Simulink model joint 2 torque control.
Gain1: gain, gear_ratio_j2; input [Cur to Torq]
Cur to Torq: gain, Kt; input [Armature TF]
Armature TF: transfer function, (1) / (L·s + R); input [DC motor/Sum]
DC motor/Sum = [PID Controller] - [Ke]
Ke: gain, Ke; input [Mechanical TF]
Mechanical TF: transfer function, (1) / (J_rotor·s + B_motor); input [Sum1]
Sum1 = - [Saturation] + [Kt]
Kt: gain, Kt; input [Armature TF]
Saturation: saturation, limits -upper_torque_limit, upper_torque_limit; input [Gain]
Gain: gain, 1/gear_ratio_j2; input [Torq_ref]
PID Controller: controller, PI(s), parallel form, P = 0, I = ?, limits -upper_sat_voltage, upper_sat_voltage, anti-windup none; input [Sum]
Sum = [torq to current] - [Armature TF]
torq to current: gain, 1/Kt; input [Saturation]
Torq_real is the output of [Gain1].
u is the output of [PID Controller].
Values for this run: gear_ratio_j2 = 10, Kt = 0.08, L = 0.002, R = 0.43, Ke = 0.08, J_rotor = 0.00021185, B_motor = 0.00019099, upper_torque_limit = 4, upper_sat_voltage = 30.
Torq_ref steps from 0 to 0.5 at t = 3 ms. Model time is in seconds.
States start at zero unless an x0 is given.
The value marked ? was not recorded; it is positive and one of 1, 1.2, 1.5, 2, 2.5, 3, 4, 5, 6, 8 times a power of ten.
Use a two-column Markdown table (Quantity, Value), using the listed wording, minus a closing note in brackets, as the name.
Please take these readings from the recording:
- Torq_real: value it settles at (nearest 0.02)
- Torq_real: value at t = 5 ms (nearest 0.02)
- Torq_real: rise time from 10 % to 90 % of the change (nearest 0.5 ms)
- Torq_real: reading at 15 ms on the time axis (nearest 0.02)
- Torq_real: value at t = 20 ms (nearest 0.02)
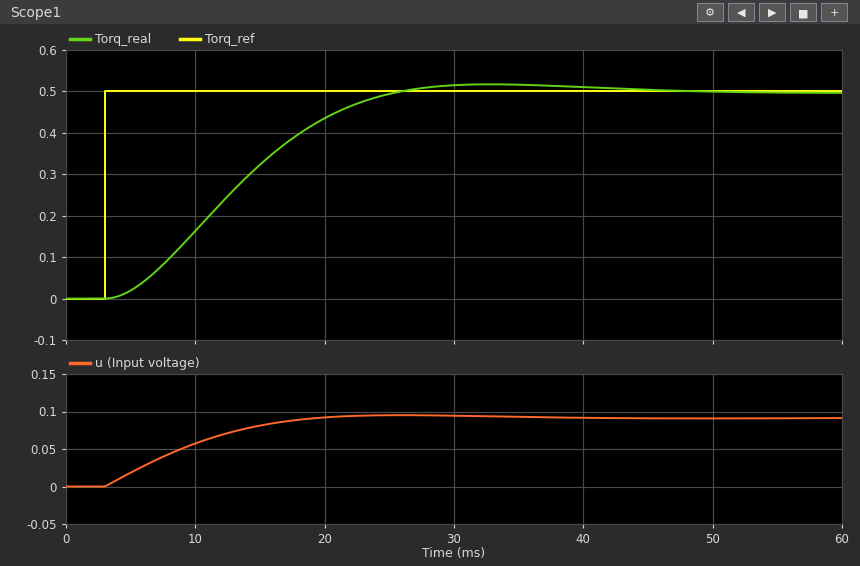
| Quantity | Value |
|---|---|
| Torq_real: value it settles at | 0.50 |
| Torq_real: value at t = 5 ms | 0.02 |
| Torq_real: rise time from 10 % to 90 % of the change | 14.5 ms |
| Torq_real: reading at 15 ms on the time axis | 0.32 |
| Torq_real: value at t = 20 ms | 0.44 |
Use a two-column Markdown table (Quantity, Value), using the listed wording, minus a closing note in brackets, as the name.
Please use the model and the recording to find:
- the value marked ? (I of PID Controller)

| Quantity | Value |
|---|---|
| the value marked ? | 15 |
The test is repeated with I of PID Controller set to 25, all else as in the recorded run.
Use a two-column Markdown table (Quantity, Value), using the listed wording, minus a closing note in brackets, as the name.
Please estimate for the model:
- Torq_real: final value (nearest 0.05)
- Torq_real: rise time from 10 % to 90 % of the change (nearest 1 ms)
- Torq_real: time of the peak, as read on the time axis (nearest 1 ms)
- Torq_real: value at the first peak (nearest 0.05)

| Quantity | Value |
|---|---|
| Torq_real: final value | 0.50 |
| Torq_real: rise time from 10 % to 90 % of the change | 12 ms |
| Torq_real: time of the peak, as read on the time axis | 28 ms |
| Torq_real: value at the first peak | 0.55 |
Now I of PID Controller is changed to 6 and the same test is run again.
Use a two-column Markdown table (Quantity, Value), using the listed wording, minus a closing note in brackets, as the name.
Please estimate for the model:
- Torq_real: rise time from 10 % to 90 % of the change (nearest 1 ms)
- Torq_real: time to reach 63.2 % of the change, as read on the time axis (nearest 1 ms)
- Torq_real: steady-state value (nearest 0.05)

| Quantity | Value |
|---|---|
| Torq_real: rise time from 10 % to 90 % of the change | 18 ms |
| Torq_real: time to reach 63.2 % of the change, as read on the time axis | 17 ms |
| Torq_real: steady-state value | 0.50 |
